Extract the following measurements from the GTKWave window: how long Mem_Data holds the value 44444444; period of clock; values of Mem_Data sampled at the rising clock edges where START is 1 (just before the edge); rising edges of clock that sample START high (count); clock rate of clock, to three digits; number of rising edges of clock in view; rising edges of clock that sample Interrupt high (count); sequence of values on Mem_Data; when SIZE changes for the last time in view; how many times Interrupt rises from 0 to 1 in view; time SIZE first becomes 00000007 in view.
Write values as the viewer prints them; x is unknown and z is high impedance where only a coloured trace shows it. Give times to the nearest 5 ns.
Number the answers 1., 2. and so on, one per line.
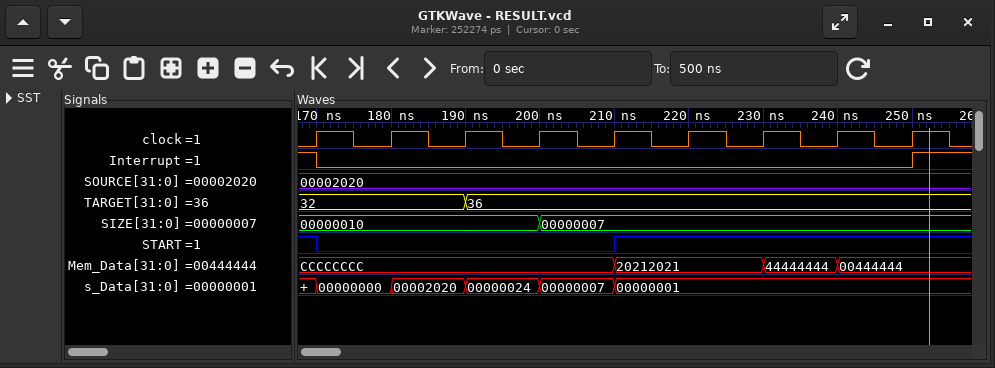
1. 10 ns
2. 10 ns
3. CCCCCCCC, 20212021, 20212021, 44444444, 00444444
4. 5
5. 100 MHz
6. 9
7. 1
8. CCCCCCCC, 20212021, 44444444, 00444444
9. 200 ns
10. 1
11. 200 ns
